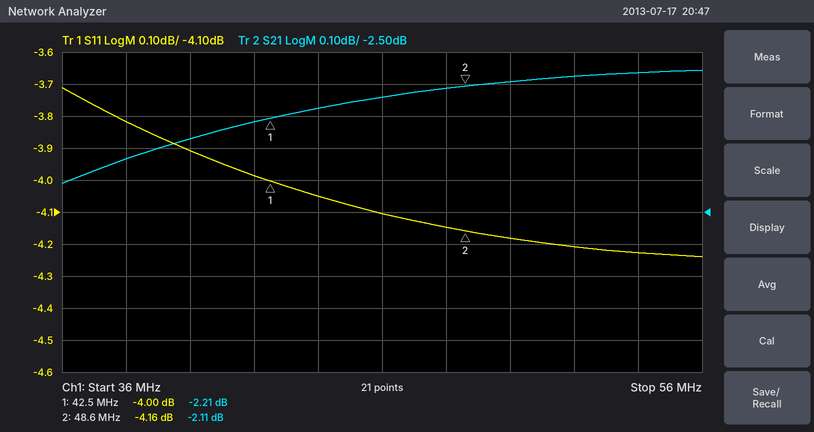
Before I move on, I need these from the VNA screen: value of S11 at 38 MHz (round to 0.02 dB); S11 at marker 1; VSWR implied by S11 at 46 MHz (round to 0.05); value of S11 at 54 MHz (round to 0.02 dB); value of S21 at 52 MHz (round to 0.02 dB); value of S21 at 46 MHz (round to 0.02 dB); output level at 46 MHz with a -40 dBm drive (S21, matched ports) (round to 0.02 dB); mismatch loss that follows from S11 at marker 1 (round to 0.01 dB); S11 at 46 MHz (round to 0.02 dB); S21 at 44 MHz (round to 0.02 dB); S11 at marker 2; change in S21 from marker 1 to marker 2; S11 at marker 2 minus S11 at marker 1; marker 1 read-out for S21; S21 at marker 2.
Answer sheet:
-3.82 dB
-4.00 dB
4.30
-4.22 dB
-2.08 dB
-2.14 dB
-42.14 dBm
2.20 dB
-4.10 dB
-2.18 dB
-4.16 dB
0.10 dB
-0.16 dB
-2.21 dB
-2.11 dB
